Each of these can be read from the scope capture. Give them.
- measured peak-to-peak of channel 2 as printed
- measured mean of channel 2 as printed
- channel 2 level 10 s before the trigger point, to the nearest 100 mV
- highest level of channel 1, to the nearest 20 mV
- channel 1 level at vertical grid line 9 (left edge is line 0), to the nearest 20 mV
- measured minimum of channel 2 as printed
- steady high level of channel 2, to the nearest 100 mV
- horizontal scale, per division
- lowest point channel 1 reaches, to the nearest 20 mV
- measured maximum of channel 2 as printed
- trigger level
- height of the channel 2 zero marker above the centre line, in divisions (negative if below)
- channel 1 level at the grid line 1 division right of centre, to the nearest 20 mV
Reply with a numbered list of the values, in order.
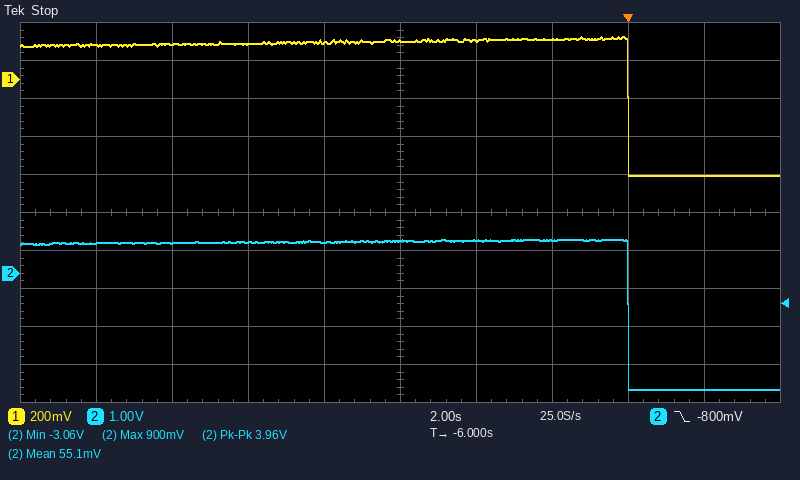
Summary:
1. 3.96 V
2. 55.1 mV
3. 800 mV
4. 220 mV
5. -500 mV
6. -3.06 V
7. 800 mV
8. 2 s
9. -500 mV
10. 900 mV
11. -800 mV
12. -1.6 div
13. 200 mV
